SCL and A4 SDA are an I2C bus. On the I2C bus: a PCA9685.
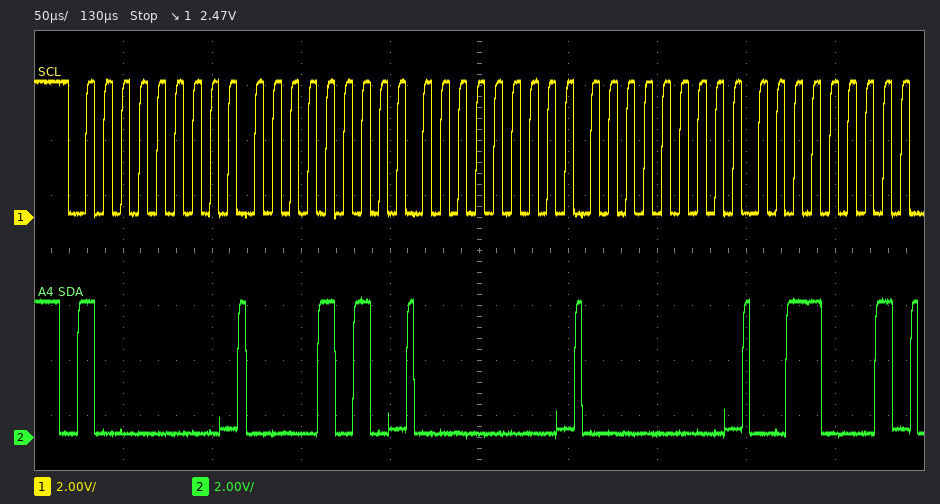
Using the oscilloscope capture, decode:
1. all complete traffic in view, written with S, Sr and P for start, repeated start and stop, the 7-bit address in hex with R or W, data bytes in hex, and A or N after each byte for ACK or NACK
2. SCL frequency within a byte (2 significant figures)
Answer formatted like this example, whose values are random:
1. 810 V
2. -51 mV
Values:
1. S 40W A 0A A 00 A 00 A 31 A
2. 100 kHz
